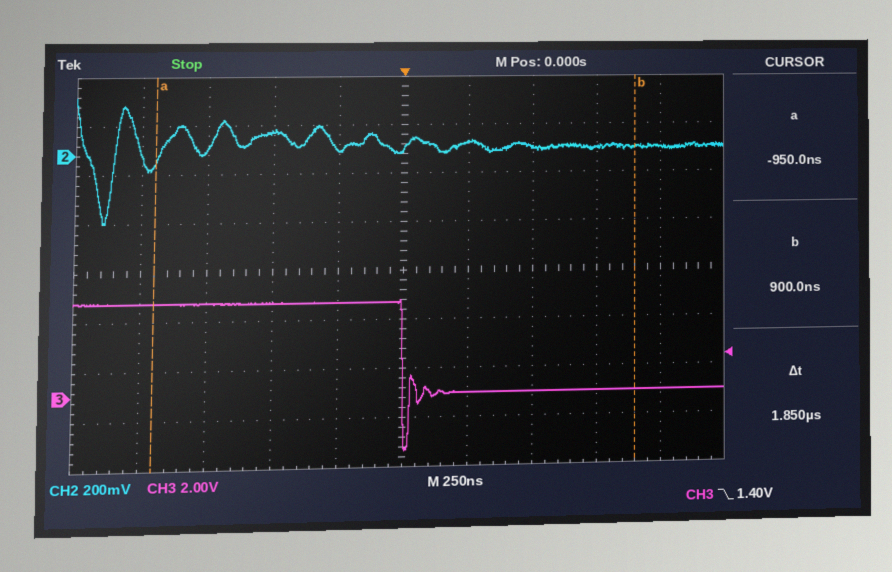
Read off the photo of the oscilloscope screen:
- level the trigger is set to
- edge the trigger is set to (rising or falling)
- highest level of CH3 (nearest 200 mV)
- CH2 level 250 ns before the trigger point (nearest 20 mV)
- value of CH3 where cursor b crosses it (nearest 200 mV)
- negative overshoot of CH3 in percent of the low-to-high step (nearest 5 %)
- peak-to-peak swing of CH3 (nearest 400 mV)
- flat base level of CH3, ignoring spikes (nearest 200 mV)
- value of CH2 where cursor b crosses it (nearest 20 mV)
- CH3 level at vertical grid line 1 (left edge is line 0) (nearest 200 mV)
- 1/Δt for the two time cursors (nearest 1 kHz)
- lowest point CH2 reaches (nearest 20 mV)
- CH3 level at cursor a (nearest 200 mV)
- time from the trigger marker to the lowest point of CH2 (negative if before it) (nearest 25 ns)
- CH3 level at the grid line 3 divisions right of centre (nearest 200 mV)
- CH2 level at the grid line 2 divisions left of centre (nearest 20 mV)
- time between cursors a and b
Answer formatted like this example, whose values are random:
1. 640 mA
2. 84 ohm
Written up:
1. 1.40 V
2. falling
3. 3.8 V
4. 20 mV
5. 0.0 V
6. 60 %
7. 6.0 V
8. 0.0 V
9. 20 mV
10. 3.8 V
11. 541 kHz
12. -280 mV
13. 3.8 V
14. -1.150 µs
15. 0.0 V
16. 100 mV
17. 1.85 µs
